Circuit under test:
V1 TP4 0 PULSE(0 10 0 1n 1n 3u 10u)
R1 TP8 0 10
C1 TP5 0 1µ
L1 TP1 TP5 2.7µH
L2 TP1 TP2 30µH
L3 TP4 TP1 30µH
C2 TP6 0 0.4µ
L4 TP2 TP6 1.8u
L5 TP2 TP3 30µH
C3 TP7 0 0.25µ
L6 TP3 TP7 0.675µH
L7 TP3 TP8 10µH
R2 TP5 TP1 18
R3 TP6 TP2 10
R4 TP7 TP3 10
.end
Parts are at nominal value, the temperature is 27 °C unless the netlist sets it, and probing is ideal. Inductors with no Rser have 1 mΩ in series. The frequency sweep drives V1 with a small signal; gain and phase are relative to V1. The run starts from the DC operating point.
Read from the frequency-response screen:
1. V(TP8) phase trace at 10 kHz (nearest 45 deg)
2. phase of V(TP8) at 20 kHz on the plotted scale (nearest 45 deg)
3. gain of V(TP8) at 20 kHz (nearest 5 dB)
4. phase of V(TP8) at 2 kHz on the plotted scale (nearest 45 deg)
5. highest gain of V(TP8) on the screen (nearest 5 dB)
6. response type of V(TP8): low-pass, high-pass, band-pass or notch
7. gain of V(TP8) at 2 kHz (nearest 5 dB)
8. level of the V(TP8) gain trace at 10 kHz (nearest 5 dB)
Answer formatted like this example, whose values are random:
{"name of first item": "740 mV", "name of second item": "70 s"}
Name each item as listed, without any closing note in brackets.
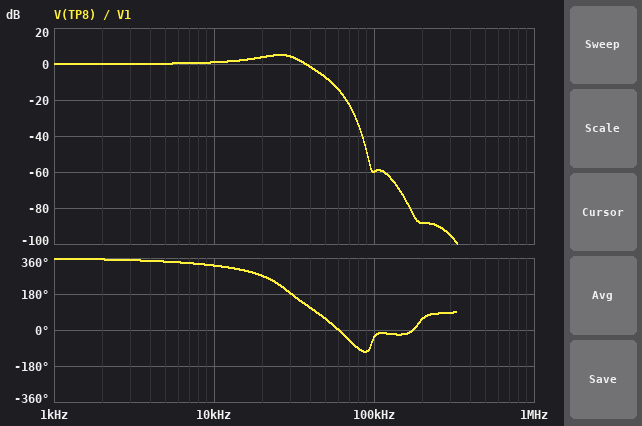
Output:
{"V(TP8) phase trace at 10 kHz": "315 deg", "phase of V(TP8) at 20 kHz on the plotted scale": "270 deg", "gain of V(TP8) at 20 kHz": "5 dB", "phase of V(TP8) at 2 kHz on the plotted scale": "360 deg", "highest gain of V(TP8) on the screen": "5 dB", "response type of V(TP8): low-pass, high-pass, band-pass or notch": "low-pass", "gain of V(TP8) at 2 kHz": "0 dB", "level of the V(TP8) gain trace at 10 kHz": "0 dB"}
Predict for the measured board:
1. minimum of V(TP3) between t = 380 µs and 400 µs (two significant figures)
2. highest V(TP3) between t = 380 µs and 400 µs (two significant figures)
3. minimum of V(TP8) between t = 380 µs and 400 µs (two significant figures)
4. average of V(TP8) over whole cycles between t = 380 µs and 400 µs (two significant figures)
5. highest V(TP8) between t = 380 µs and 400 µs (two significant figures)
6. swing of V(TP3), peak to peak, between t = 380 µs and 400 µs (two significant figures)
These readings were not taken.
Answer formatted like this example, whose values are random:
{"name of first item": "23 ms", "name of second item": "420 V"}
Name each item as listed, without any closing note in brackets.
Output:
{"minimum of V(TP3) between t = 380 µs and 400 µs": "3.0 V", "highest V(TP3) between t = 380 µs and 400 µs": "3.0 V", "minimum of V(TP8) between t = 380 µs and 400 µs": "3.0 V", "average of V(TP8) over whole cycles between t = 380 µs and 400 µs": "3.0 V", "highest V(TP8) between t = 380 µs and 400 µs": "3.0 V", "swing of V(TP3), peak to peak, between t = 380 µs and 400 µs": "12 mV"}
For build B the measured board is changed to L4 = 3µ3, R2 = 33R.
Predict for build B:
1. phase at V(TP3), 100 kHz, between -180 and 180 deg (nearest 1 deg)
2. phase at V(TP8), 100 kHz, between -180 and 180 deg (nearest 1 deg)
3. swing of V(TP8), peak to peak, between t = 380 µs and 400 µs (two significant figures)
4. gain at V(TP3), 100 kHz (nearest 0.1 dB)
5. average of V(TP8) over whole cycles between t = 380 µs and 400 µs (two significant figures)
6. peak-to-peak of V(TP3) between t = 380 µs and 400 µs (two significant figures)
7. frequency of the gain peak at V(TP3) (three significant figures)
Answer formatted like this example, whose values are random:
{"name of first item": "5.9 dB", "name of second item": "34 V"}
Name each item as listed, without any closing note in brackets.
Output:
{"phase at V(TP3), 100 kHz, between -180 and 180 deg": "24 deg", "phase at V(TP8), 100 kHz, between -180 and 180 deg": "-8 deg", "swing of V(TP8), peak to peak, between t = 380 µs and 400 µs": "4.8 mV", "gain at V(TP3), 100 kHz": "-65.7 dB", "average of V(TP8) over whole cycles between t = 380 µs and 400 µs": "3.0 V", "peak-to-peak of V(TP3) between t = 380 µs and 400 µs": "6.0 mV", "frequency of the gain peak at V(TP3)": "25.9 kHz"}
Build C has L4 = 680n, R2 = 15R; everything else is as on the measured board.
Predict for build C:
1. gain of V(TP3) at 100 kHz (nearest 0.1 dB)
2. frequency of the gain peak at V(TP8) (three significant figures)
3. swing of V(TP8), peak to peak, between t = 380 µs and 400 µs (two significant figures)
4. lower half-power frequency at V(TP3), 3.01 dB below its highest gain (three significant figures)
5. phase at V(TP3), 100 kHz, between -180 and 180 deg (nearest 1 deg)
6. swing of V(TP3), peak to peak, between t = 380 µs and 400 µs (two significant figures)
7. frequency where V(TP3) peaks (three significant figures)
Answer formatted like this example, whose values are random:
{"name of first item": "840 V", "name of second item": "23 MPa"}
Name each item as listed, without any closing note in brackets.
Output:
{"gain of V(TP3) at 100 kHz": "-54.3 dB", "frequency of the gain peak at V(TP8)": "26.1 kHz", "swing of V(TP8), peak to peak, between t = 380 µs and 400 µs": "17 mV", "lower half-power frequency at V(TP3), 3.01 dB below its highest gain": "14.9 kHz", "phase at V(TP3), 100 kHz, between -180 and 180 deg": "-11 deg", "swing of V(TP3), peak to peak, between t = 380 µs and 400 µs": "20 mV", "frequency where V(TP3) peaks": "26.2 kHz"}
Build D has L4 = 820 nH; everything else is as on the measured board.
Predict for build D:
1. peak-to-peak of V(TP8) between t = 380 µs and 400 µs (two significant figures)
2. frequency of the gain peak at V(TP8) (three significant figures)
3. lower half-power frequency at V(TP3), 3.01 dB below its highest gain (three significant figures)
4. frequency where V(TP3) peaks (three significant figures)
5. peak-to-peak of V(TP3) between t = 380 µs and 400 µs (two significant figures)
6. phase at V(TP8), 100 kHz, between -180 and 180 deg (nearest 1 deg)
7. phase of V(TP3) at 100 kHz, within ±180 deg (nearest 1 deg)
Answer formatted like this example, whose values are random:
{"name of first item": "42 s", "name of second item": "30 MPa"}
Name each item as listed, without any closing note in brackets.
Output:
{"peak-to-peak of V(TP8) between t = 380 µs and 400 µs": "14 mV", "frequency of the gain peak at V(TP8)": "26.1 kHz", "lower half-power frequency at V(TP3), 3.01 dB below its highest gain": "14.9 kHz", "frequency where V(TP3) peaks": "26.2 kHz", "peak-to-peak of V(TP3) between t = 380 µs and 400 µs": "17 mV", "phase at V(TP8), 100 kHz, between -180 and 180 deg": "-38 deg", "phase of V(TP3) at 100 kHz, within ±180 deg": "-6 deg"}
